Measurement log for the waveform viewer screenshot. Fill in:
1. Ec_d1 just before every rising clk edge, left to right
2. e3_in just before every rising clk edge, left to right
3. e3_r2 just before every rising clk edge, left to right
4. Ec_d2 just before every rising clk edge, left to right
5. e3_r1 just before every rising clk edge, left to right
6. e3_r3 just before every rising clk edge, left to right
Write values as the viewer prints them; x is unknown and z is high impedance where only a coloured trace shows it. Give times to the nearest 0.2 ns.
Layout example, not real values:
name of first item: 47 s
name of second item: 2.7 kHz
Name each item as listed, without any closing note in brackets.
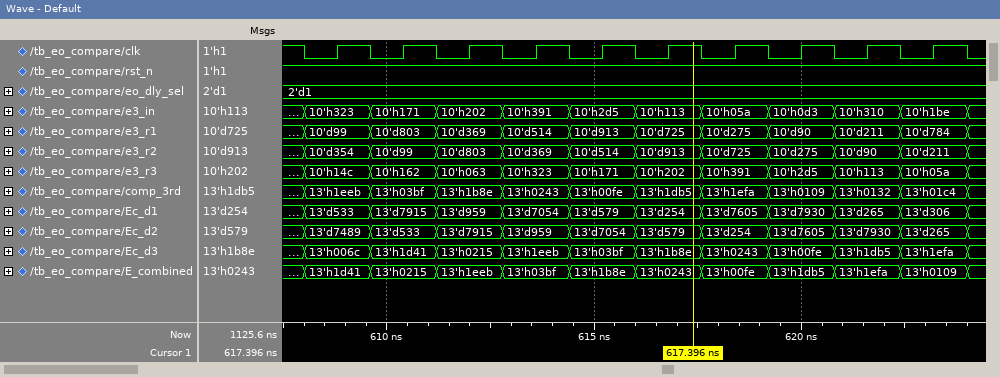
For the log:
Ec_d1 just before every rising clk edge, left to right: 13'd533, 13'd7915, 13'd959, 13'd7054, 13'd579, 13'd254, 13'd7605, 13'd7930, 13'd265, 13'd306
e3_in just before every rising clk edge, left to right: 10'h323, 10'h171, 10'h202, 10'h391, 10'h2d5, 10'h113, 10'h05a, 10'h0d3, 10'h310, 10'h1be
e3_r2 just before every rising clk edge, left to right: 10'd354, 10'd99, 10'd803, 10'd369, 10'd514, 10'd913, 10'd725, 10'd275, 10'd90, 10'd211
Ec_d2 just before every rising clk edge, left to right: 13'd7489, 13'd533, 13'd7915, 13'd959, 13'd7054, 13'd579, 13'd254, 13'd7605, 13'd7930, 13'd265
e3_r1 just before every rising clk edge, left to right: 10'd99, 10'd803, 10'd369, 10'd514, 10'd913, 10'd725, 10'd275, 10'd90, 10'd211, 10'd784
e3_r3 just before every rising clk edge, left to right: 10'h14c, 10'h162, 10'h063, 10'h323, 10'h171, 10'h202, 10'h391, 10'h2d5, 10'h113, 10'h05a
